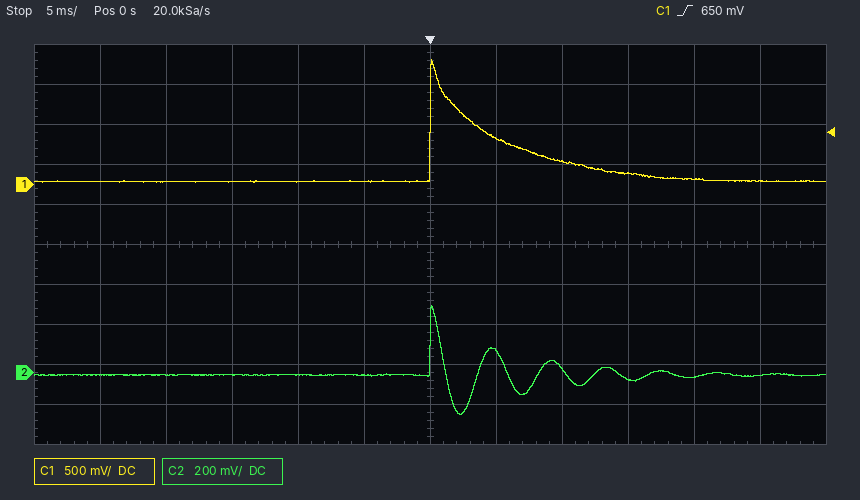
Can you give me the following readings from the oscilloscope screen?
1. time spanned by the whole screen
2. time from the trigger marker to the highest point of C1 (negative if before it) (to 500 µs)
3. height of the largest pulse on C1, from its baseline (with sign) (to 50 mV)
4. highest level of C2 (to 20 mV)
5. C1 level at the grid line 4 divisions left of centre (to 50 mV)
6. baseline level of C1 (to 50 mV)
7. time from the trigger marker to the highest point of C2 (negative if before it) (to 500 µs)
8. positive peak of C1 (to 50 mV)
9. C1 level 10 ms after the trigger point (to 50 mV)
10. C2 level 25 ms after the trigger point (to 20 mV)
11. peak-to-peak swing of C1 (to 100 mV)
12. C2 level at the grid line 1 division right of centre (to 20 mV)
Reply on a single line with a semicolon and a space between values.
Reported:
60 ms; 0.0 ms; +1.50 V; 340 mV; 50 mV; 50 mV; 0.0 ms; 1.55 V; 300 mV; -20 mV; 1.50 V; 100 mV
